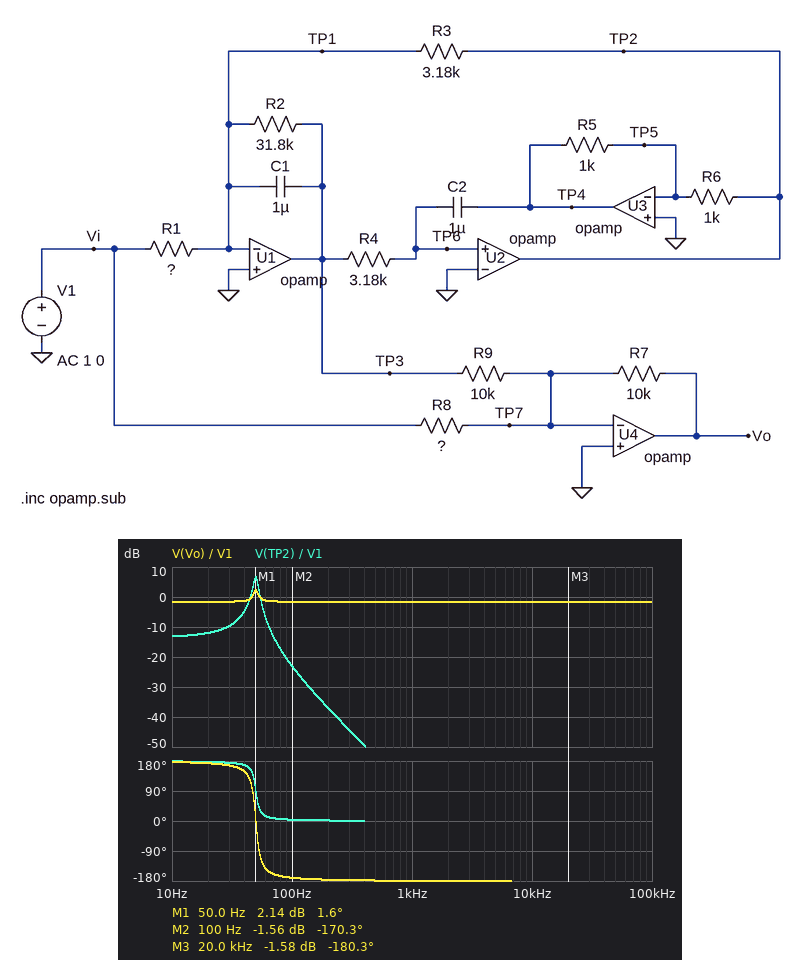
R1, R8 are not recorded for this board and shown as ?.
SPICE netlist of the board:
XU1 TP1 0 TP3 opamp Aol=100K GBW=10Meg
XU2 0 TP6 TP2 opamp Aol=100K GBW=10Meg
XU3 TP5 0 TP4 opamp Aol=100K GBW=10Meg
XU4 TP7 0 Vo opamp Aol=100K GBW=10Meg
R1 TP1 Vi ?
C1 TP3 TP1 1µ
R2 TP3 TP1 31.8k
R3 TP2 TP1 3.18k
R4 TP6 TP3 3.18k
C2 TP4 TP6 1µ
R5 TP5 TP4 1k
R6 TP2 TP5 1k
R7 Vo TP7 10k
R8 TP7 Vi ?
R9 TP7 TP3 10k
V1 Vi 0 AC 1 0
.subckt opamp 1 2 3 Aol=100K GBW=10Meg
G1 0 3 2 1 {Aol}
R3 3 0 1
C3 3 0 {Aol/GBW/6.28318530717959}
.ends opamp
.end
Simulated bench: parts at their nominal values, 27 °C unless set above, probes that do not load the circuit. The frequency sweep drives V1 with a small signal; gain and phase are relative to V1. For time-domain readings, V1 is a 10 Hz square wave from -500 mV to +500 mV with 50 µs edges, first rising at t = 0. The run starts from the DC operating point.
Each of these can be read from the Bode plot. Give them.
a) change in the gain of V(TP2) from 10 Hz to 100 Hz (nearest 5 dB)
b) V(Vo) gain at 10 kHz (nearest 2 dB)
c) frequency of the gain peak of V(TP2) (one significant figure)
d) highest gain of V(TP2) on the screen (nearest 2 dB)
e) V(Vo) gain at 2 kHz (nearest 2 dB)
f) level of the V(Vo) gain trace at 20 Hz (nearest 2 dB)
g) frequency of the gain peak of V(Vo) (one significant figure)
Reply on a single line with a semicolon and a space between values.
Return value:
-10 dB; -2 dB; 50 Hz; 6 dB; -2 dB; -2 dB; 50 Hz
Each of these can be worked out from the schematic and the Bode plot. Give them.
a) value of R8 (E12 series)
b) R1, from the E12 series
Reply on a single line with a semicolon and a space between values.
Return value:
12 kΩ; 15 kΩ
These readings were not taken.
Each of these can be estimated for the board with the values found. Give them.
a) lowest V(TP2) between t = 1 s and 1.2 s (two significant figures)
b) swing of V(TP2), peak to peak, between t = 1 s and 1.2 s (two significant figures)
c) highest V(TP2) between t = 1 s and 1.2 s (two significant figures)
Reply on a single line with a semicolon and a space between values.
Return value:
-440 mV; 880 mV; 440 mV
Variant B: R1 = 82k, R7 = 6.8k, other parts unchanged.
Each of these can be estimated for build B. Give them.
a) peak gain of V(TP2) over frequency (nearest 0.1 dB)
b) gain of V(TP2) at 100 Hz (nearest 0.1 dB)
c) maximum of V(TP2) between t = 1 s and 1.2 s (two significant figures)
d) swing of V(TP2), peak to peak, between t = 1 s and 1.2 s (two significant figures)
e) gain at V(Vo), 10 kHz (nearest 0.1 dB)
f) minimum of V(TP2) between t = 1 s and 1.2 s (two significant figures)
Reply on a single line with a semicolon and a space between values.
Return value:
-8.2 dB; -37.8 dB; 80 mV; 160 mV; -4.9 dB; -80 mV
